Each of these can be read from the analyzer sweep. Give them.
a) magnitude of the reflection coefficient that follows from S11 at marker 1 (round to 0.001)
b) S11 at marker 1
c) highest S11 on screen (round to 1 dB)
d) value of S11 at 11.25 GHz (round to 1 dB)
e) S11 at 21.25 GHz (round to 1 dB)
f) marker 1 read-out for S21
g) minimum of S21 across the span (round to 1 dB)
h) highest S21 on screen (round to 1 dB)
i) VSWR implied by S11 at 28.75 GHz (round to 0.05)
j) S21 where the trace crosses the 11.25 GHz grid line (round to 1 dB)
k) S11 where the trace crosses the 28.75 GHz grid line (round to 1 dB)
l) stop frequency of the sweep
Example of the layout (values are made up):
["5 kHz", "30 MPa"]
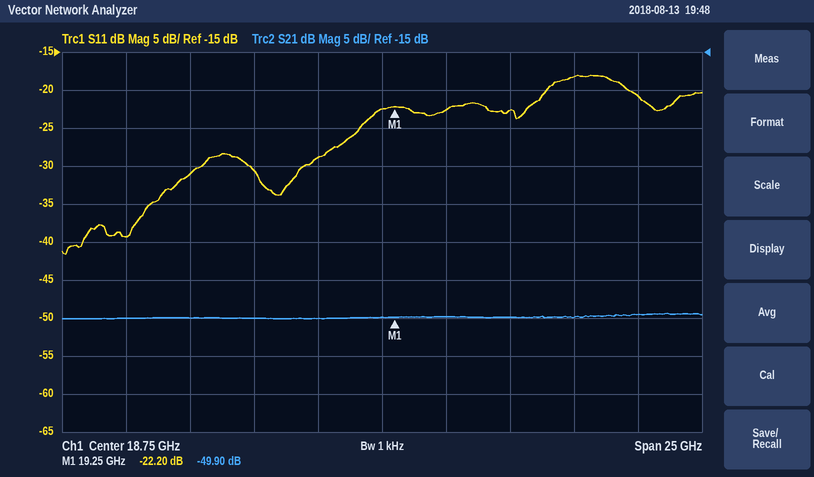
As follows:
["0.078", "-22.20 dB", "-18 dB", "-31 dB", "-23 dB", "-49.90 dB", "-50 dB", "-49 dB", "1.20", "-50 dB", "-21 dB", "31.25 GHz"]
